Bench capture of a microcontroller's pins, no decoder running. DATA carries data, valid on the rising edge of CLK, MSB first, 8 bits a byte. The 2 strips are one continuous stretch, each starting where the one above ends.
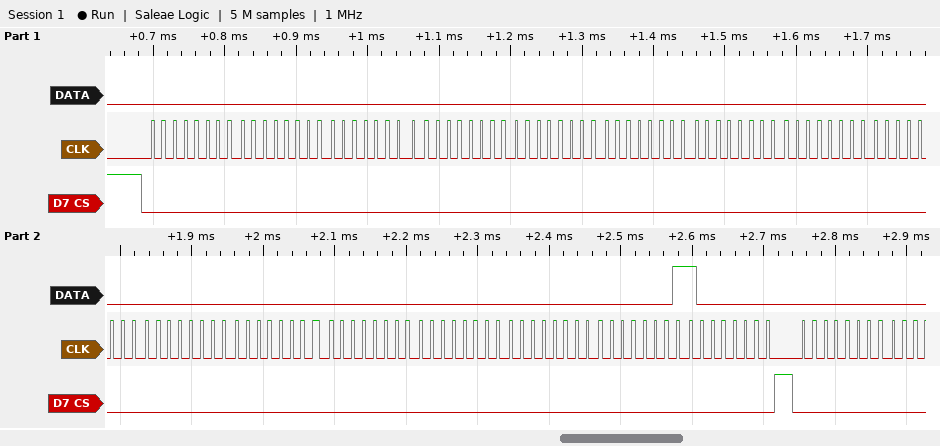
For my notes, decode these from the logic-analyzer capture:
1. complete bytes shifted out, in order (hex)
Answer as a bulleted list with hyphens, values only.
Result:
- 0x00 0x00 0x00 0x00 0x00 0x00 0x00 0x00 0x00 0x00 0x00 0x00 0x00 0x00 0x01 0x80 0x00
